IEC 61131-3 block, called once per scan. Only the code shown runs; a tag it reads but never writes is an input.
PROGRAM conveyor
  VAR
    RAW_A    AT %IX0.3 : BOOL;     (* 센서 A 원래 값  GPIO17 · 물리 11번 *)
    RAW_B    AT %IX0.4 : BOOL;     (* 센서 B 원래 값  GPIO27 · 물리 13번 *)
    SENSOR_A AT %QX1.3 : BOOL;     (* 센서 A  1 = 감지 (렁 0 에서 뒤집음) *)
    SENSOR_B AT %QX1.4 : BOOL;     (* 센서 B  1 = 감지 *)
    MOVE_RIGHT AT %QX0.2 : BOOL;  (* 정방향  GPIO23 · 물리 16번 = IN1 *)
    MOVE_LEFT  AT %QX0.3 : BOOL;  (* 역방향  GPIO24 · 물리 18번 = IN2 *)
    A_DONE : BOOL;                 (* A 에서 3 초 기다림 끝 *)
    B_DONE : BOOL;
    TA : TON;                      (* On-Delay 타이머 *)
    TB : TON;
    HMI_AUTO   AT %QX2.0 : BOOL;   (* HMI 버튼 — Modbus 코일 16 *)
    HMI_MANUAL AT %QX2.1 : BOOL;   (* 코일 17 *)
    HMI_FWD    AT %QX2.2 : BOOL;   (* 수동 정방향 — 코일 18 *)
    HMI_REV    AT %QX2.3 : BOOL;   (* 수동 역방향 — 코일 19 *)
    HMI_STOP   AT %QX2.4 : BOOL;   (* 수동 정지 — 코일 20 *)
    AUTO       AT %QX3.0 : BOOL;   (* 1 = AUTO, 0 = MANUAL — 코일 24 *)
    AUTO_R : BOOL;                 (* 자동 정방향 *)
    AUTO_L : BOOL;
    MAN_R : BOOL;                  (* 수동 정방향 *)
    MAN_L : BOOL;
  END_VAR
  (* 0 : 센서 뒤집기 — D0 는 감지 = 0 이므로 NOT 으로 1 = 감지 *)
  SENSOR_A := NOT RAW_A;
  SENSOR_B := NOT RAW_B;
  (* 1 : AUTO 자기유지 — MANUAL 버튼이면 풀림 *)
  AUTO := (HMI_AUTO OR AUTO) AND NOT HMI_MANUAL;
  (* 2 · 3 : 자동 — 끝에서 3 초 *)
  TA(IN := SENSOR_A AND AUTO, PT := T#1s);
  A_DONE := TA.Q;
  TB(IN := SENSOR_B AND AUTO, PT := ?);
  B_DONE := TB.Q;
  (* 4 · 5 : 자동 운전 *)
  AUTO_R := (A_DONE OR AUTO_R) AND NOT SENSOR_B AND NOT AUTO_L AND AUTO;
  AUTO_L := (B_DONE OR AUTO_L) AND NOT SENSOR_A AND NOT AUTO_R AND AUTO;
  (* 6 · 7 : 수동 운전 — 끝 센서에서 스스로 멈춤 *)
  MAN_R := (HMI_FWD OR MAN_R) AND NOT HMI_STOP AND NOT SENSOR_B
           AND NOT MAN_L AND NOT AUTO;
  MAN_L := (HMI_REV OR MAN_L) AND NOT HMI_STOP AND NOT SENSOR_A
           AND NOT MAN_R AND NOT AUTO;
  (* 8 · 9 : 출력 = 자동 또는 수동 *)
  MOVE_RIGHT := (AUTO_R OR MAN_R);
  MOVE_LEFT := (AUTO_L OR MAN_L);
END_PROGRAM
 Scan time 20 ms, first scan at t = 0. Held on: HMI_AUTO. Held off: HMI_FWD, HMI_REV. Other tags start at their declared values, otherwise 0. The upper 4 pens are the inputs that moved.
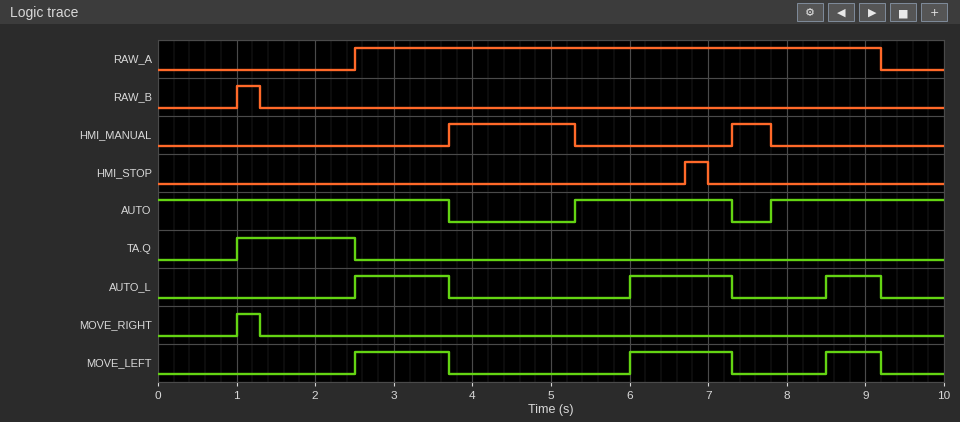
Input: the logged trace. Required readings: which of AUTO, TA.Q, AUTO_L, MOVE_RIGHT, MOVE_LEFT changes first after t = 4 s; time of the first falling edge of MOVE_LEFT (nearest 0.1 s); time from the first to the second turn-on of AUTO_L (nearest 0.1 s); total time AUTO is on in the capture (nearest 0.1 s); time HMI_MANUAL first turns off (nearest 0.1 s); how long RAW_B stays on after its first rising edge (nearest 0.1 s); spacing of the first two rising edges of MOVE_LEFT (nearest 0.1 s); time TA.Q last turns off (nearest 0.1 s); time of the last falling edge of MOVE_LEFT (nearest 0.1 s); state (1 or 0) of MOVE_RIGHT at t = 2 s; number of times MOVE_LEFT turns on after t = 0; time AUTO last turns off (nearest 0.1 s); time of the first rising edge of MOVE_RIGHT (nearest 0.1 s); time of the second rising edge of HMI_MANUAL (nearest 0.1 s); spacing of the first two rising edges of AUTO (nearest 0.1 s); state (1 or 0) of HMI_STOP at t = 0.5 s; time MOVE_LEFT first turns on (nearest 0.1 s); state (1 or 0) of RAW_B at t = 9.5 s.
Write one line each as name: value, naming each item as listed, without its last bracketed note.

which of AUTO, TA.Q, AUTO_L, MOVE_RIGHT, MOVE_LEFT changes first after t = 4 s: AUTO
time of the first falling edge of MOVE_LEFT: 3.7 s
time from the first to the second turn-on of AUTO_L: 3.5 s
total time AUTO is on in the capture: 7.9 s
time HMI_MANUAL first turns off: 5.3 s
how long RAW_B stays on after its first rising edge: 0.3 s
spacing of the first two rising edges of MOVE_LEFT: 3.5 s
time TA.Q last turns off: 2.5 s
time of the last falling edge of MOVE_LEFT: 9.2 s
state (1 or 0) of MOVE_RIGHT at t = 2 s: 0
number of times MOVE_LEFT turns on after t = 0: 3
time AUTO last turns off: 7.3 s
time of the first rising edge of MOVE_RIGHT: 1.0 s
time of the second rising edge of HMI_MANUAL: 7.3 s
spacing of the first two rising edges of AUTO: 2.5 s
state (1 or 0) of HMI_STOP at t = 0.5 s: 0
time MOVE_LEFT first turns on: 2.5 s
state (1 or 0) of RAW_B at t = 9.5 s: 0
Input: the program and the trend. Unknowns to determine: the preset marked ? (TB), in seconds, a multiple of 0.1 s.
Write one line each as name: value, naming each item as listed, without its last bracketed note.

the preset marked ? (TB), in seconds, a multiple of 0.1 s: 0.7 s
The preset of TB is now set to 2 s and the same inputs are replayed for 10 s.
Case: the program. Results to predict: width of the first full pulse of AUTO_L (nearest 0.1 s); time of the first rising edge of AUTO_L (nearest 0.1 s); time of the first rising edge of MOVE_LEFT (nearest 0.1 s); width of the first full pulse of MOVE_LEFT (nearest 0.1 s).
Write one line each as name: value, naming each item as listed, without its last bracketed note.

width of the first full pulse of AUTO_L: 0.4 s
time of the first rising edge of AUTO_L: 3.3 s
time of the first rising edge of MOVE_LEFT: 3.3 s
width of the first full pulse of MOVE_LEFT: 0.4 s
